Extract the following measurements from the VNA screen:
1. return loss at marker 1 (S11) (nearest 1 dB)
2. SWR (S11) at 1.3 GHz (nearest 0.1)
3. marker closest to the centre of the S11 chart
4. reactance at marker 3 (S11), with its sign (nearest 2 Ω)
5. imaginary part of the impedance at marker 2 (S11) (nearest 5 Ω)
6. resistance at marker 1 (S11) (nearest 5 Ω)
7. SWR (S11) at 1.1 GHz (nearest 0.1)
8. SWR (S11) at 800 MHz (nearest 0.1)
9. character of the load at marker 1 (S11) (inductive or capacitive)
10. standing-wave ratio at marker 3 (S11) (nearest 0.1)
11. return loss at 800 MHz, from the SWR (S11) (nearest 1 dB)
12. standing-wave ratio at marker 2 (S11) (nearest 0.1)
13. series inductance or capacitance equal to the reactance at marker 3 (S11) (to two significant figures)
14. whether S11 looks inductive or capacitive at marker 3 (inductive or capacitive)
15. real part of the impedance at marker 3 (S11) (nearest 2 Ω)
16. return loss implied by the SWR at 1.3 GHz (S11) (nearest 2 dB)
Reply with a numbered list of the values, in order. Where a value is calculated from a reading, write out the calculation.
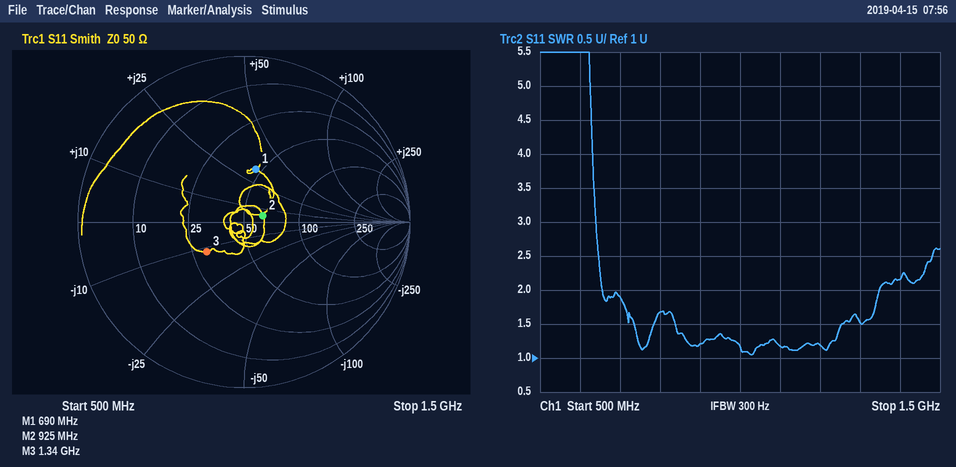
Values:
1. 10 dB
2. 1.5
3. marker 2
4. -12 Ω
5. +5 Ω
6. 45 Ω
7. 1.2
8. 1.7
9. inductive
10. 1.8
11. −20 log10((1.7 − 1)/(1.7 + 1)) ≈ 12 dB
12. 1.3
13. C = 1/(2π × 1.34 GHz × 12 Ω) ≈ 10 pF
14. capacitive
15. 30 Ω
16. −20 log10((1.5 − 1)/(1.5 + 1)) ≈ 14 dB
